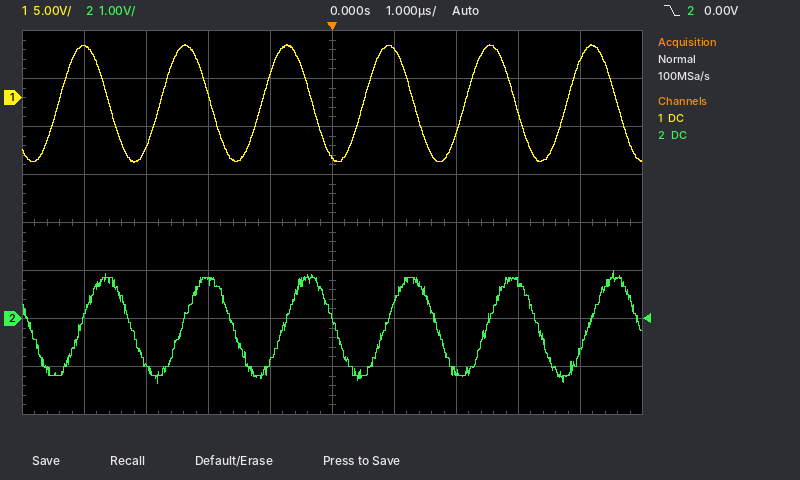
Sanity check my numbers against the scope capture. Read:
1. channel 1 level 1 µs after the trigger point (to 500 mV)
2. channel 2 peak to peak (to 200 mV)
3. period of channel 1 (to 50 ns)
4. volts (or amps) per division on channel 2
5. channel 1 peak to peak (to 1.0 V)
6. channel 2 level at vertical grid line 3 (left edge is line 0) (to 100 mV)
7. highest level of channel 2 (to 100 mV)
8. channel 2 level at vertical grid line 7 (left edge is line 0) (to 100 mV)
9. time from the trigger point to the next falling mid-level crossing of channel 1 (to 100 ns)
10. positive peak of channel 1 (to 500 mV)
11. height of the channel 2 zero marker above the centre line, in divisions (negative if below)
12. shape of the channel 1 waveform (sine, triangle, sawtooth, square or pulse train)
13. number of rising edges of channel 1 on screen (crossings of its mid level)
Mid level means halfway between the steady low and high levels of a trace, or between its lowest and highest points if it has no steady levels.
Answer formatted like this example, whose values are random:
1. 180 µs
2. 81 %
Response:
1. 5.0 V
2. 2.4 V
3. 1.65 µs
4. 1 V
5. 12.0 V
6. 800 mV
7. 1.0 V
8. -1.1 V
9. 1.3 µs
10. 5.5 V
11. -2.0 div
12. sine
13. 6
